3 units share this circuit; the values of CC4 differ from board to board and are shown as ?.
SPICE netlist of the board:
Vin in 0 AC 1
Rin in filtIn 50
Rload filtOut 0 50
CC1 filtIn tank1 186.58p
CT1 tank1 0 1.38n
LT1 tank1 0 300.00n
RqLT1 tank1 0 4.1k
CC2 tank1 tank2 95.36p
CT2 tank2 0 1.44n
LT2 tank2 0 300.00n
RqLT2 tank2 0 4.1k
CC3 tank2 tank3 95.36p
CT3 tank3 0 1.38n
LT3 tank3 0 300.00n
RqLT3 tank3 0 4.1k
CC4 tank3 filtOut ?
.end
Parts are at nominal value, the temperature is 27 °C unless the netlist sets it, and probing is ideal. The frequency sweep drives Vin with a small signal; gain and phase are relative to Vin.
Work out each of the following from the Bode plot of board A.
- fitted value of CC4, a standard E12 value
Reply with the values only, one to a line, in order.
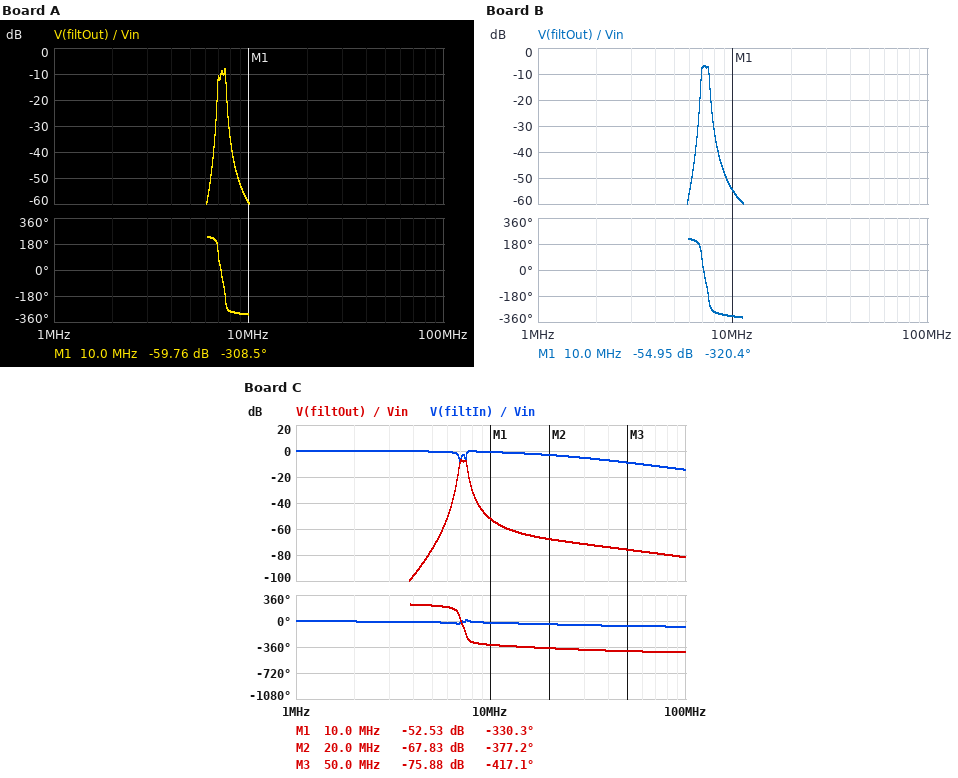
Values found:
100 pF
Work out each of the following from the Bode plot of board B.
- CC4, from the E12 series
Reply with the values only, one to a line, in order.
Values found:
220 pF
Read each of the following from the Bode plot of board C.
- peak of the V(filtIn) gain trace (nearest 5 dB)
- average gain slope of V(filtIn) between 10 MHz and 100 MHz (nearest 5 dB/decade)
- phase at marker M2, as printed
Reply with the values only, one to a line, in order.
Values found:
0 dB
-15 dB/decade
-377.2 deg
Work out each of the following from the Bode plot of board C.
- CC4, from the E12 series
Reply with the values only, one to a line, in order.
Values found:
390 pF
